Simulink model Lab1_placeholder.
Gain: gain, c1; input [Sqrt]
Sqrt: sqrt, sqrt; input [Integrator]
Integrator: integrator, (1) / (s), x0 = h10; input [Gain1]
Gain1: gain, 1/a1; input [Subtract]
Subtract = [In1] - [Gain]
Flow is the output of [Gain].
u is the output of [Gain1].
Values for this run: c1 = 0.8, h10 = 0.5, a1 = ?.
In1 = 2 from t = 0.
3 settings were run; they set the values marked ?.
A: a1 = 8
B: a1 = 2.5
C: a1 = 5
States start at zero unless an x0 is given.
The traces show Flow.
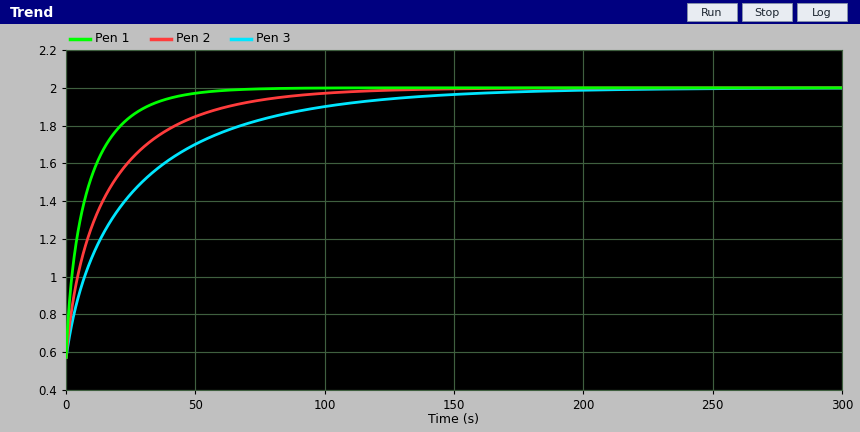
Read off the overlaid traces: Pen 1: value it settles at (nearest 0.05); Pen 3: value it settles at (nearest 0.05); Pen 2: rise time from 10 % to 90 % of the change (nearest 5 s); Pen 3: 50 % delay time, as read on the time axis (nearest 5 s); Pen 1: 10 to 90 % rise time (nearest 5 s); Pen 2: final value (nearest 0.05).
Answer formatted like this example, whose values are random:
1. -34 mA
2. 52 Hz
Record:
1. 2.00
2. 2.00
3. 50 s
4. 15 s
5. 25 s
6. 2.00
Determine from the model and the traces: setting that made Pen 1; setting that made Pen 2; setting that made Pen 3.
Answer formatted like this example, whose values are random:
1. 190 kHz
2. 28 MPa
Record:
1. B
2. C
3. A
